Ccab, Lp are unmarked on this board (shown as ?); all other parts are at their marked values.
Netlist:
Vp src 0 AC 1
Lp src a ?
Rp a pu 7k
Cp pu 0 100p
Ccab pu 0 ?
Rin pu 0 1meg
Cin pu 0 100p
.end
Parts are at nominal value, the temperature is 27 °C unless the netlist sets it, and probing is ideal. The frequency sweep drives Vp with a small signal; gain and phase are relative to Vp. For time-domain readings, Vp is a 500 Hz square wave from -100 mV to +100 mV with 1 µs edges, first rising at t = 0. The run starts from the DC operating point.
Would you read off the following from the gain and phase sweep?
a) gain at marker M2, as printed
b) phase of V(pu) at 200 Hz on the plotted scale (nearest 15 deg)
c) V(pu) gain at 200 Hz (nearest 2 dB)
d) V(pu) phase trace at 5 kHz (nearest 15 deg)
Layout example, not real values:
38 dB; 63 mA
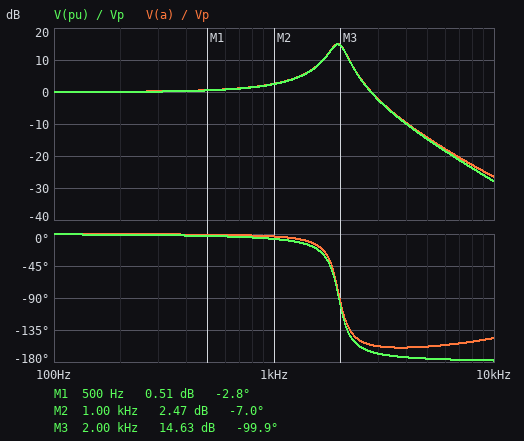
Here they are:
2.47 dB; 0 deg; 0 dB; -180 deg
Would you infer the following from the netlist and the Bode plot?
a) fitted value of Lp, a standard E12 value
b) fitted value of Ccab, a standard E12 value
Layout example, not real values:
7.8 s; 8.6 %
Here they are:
4.7 H; 1.2 nF
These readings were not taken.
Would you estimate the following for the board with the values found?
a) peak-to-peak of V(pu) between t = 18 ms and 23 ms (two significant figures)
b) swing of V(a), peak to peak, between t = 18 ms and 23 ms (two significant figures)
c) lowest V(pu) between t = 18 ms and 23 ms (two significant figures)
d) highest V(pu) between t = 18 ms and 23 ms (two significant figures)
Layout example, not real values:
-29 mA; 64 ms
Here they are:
430 mV; 430 mV; -210 mV; 210 mV
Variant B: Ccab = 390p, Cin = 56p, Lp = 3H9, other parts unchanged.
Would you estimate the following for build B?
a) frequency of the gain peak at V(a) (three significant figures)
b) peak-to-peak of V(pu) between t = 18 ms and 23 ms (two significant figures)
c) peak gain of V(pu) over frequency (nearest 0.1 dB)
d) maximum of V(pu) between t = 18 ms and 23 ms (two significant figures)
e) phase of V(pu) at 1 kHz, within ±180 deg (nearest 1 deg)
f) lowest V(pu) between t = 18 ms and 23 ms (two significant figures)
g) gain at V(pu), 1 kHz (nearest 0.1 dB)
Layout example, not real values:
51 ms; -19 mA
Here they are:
3.44 kHz; 560 mV; 15.5 dB; 280 mV; -3 deg; -280 mV; 0.7 dB
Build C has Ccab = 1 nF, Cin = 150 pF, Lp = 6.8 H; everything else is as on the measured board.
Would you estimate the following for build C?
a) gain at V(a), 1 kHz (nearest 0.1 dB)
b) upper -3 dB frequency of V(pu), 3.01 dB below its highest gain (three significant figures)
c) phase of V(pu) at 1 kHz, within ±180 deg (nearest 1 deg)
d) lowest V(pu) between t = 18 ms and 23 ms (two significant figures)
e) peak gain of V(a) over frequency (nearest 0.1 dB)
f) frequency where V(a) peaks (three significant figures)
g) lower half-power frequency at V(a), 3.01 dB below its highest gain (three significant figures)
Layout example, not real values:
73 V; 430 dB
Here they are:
3.4 dB; 1.86 kHz; -8 deg; -250 mV; 15.6 dB; 1.72 kHz; 1.57 kHz
